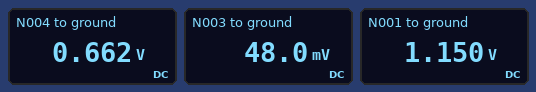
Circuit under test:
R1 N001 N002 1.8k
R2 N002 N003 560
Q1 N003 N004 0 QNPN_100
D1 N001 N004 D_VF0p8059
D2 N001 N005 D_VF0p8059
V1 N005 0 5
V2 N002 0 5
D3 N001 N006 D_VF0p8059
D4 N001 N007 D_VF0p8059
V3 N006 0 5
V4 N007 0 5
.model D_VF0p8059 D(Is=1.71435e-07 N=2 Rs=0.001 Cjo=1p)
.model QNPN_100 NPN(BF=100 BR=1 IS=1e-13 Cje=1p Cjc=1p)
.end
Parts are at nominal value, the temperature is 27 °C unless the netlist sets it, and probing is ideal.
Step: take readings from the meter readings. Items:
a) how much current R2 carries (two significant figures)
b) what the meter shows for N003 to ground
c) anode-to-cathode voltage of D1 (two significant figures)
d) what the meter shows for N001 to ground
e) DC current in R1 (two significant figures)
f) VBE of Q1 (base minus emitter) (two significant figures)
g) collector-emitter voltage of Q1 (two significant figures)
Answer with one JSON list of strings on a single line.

["8.8 mA", "48.0 mV", "490 mV", "1.150 V", "2.1 mA", "660 mV", "48 mV"]
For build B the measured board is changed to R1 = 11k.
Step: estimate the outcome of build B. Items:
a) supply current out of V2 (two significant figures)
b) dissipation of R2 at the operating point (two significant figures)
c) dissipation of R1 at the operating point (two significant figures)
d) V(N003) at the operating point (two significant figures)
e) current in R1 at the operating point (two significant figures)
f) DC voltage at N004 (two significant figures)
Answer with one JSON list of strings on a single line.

["9.1 mA", "43 mW", "1.4 mW", "92 mV", "360 µA", "650 mV"]
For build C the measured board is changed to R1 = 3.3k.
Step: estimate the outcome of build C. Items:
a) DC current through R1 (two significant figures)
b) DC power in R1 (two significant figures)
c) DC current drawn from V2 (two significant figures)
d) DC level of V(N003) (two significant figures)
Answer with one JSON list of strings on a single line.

["1.2 mA", "4.6 mW", "10 mA", "60 mV"]
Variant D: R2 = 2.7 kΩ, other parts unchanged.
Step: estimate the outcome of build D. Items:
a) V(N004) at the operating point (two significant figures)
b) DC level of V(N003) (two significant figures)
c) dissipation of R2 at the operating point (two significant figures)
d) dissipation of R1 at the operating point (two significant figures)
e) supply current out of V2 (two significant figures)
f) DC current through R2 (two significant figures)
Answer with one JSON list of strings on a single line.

["640 mV", "27 mV", "9.2 mW", "8.3 mW", "4.0 mA", "1.8 mA"]
